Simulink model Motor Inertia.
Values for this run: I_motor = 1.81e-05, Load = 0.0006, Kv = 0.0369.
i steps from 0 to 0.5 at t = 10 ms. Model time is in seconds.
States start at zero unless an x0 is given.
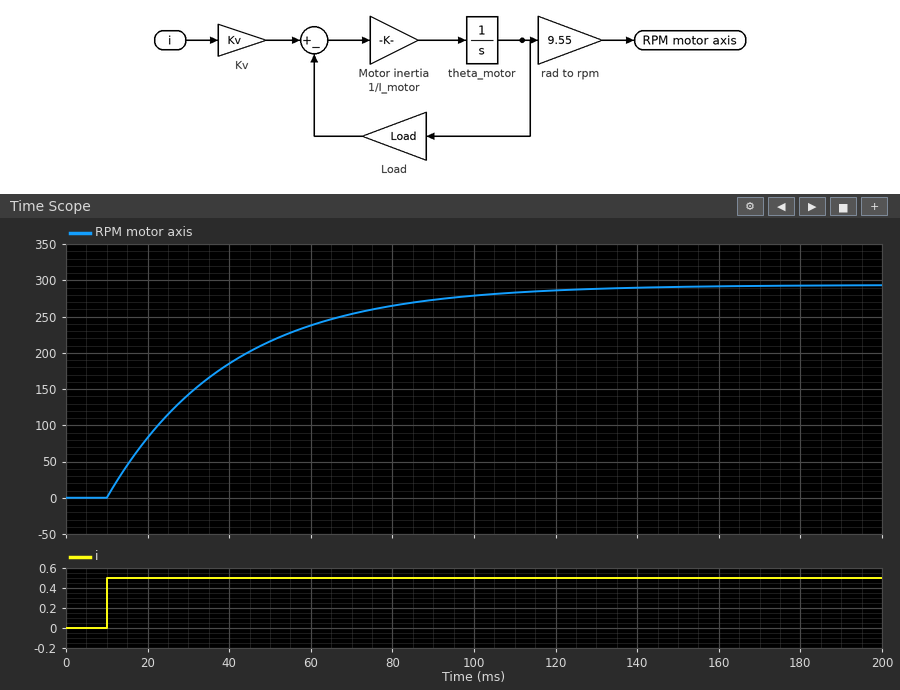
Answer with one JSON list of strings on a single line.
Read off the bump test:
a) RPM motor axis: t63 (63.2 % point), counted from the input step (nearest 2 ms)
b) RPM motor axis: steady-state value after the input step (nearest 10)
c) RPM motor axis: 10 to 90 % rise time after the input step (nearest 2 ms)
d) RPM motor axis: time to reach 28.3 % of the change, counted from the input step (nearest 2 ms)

["30 ms", "290", "66 ms", "10 ms"]
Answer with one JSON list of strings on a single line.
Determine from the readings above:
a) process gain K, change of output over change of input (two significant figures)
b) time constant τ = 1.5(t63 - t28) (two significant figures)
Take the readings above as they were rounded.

["580", "30 ms"]
